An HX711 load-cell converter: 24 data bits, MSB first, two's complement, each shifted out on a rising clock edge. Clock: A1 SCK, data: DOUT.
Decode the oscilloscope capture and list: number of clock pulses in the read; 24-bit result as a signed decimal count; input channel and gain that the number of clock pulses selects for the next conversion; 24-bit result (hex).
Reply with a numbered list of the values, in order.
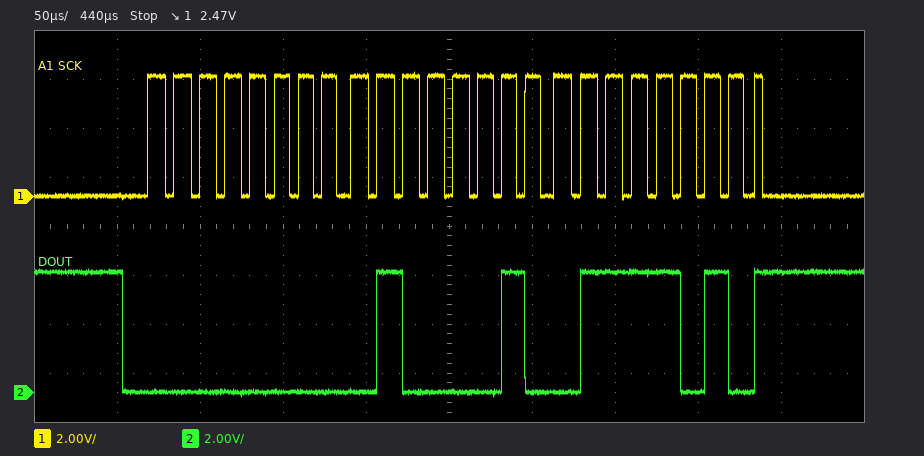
1. 25
2. 17018
3. channel A, gain 128
4. 0x00427A
